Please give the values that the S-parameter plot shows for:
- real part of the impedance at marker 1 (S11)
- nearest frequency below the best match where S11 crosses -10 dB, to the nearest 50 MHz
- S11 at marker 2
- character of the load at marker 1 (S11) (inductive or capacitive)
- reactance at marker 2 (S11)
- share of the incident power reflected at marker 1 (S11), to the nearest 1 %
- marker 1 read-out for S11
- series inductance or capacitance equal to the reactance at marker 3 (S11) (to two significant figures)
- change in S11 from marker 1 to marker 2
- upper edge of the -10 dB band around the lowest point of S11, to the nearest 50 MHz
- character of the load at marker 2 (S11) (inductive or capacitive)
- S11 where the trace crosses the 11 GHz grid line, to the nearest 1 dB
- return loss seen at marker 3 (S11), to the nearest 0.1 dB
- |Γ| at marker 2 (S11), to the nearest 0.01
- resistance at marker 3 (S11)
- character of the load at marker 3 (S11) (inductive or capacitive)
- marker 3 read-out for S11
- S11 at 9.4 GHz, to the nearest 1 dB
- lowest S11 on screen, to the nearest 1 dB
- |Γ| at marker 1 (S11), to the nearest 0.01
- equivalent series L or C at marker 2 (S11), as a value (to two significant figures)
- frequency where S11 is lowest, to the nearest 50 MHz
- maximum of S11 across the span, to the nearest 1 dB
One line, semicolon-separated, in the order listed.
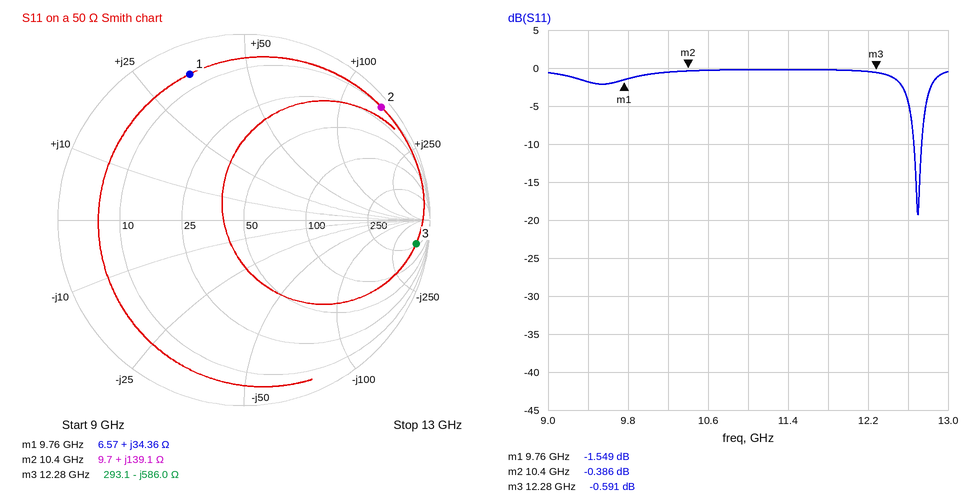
6.57 Ω; 12.65 GHz; -0.386 dB; inductive; +139.1 Ω; 70 %; -1.549 dB; 22 fF; 1.163 dB; 12.75 GHz; inductive; 0 dB; 0.6 dB; 0.96; 293.1 Ω; capacitive; -0.591 dB; -2 dB; -19 dB; 0.84; 2.1 nH; 12.70 GHz; 0 dB
